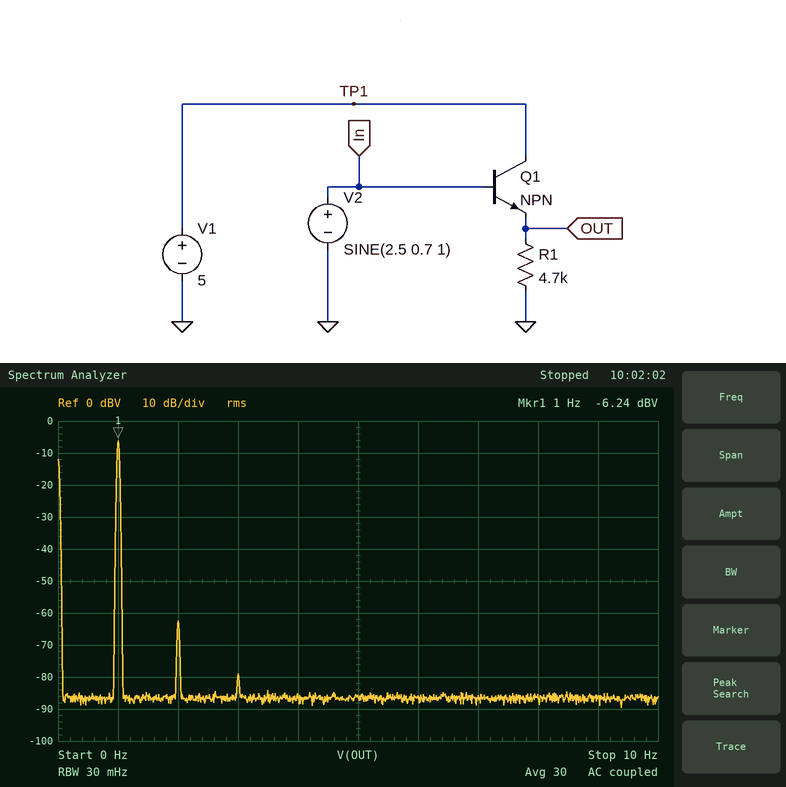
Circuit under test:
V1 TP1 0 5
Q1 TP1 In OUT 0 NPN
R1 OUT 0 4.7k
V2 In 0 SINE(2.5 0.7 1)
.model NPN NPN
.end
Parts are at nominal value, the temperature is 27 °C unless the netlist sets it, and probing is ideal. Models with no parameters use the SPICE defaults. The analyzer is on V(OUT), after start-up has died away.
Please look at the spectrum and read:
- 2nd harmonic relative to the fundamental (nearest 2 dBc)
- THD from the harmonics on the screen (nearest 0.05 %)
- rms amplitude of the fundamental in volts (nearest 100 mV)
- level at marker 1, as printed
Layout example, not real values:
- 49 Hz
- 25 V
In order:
- -56 dBc
- 0.15 %
- 500 mV
- -6.24 dBV
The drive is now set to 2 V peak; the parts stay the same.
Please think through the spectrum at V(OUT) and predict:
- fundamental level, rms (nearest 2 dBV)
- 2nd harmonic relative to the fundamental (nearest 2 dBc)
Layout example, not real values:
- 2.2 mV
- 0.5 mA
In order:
- 2 dBV
- -32 dBc
